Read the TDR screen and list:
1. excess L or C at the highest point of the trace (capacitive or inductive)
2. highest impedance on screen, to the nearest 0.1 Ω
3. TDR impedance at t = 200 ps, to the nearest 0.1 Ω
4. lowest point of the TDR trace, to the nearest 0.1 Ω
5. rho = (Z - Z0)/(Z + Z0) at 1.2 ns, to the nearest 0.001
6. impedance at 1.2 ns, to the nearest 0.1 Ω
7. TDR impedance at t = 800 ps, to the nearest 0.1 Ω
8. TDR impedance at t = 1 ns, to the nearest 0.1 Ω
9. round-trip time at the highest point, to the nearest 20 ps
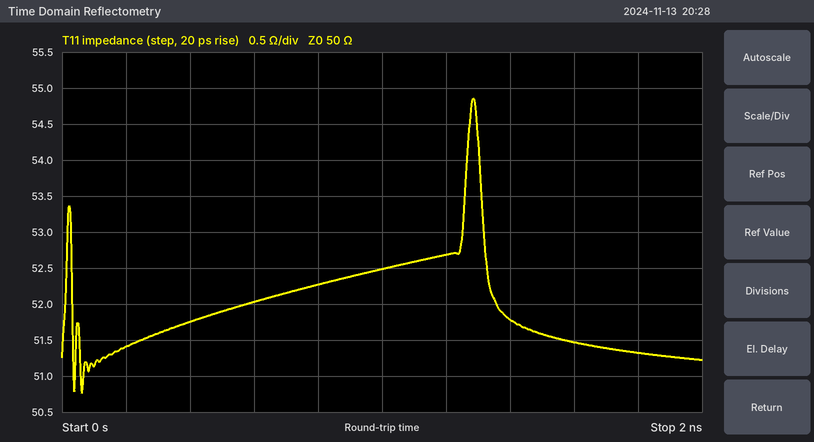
inductive
54.9 Ω
51.4 Ω
50.8 Ω
+0.026
52.7 Ω
52.3 Ω
52.5 Ω
1.28 ns
